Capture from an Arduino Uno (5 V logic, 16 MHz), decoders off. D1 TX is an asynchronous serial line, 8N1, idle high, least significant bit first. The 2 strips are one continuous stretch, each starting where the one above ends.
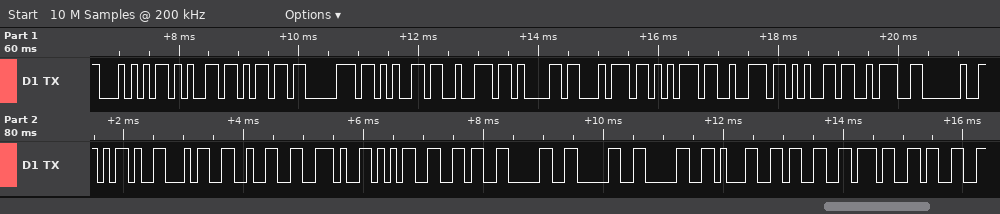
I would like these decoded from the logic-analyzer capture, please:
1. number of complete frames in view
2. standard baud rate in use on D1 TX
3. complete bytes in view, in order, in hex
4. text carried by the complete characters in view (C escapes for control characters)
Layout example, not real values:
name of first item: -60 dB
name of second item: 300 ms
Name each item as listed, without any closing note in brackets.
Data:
number of complete frames in view: 26
standard baud rate in use on D1 TX: 9600 baud
complete bytes in view, in order, in hex: 54 65 6D 70 65 72 61 74 75 72 65 3A 20 2D 34 32 2E 35 36 30 30 30 31 33 37 33
text carried by the complete characters in view: "Temperature: -42.560001373"
